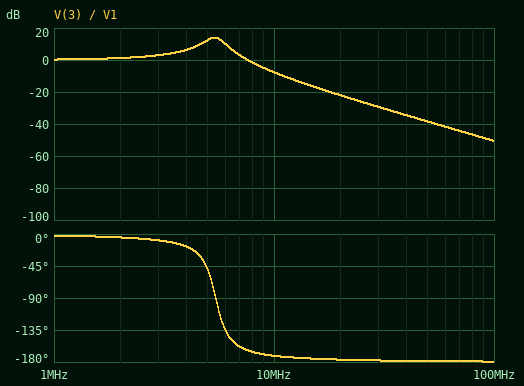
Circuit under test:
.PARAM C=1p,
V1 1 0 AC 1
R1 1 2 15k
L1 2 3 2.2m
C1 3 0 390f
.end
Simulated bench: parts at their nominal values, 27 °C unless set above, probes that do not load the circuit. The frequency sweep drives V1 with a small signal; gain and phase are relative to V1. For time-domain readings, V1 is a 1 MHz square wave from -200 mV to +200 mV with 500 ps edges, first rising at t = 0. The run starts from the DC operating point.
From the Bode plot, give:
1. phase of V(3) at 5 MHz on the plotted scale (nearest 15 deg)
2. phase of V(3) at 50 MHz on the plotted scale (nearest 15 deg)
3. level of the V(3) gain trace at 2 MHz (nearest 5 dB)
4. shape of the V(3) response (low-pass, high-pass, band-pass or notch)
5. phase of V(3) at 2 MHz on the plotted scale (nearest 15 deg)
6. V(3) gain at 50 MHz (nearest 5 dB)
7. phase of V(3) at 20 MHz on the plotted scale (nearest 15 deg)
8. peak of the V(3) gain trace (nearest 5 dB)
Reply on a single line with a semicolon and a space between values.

-45 deg; -180 deg; 0 dB; low-pass; 0 deg; -40 dB; -180 deg; 15 dB
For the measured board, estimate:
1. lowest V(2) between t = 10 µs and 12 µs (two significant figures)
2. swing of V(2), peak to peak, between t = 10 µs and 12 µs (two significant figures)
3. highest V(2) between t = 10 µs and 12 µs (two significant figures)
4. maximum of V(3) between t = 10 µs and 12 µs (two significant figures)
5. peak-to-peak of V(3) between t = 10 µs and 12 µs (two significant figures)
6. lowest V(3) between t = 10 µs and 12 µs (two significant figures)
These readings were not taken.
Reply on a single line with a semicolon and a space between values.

-250 mV; 510 mV; 250 mV; 510 mV; 1.0 V; -510 mV
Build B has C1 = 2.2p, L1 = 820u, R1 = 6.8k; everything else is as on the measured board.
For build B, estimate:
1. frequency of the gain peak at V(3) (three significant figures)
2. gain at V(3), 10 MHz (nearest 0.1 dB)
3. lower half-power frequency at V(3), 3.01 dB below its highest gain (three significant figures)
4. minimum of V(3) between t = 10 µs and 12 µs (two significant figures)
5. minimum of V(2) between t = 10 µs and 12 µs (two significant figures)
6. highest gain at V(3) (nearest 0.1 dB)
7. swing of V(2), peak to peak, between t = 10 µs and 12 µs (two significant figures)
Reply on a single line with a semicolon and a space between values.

3.63 MHz; -15.8 dB; 2.88 MHz; -420 mV; -260 mV; 9.2 dB; 520 mV
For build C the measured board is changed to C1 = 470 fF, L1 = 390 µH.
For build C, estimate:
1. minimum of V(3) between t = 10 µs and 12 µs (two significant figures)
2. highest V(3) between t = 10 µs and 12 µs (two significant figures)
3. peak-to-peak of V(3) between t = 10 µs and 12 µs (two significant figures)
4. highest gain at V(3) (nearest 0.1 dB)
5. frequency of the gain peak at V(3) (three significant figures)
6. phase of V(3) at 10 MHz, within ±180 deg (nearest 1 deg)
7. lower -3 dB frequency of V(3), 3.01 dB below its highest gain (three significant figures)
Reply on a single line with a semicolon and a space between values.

-370 mV; 370 mV; 740 mV; 6.0 dB; 10.9 MHz; -58 deg; 7.07 MHz
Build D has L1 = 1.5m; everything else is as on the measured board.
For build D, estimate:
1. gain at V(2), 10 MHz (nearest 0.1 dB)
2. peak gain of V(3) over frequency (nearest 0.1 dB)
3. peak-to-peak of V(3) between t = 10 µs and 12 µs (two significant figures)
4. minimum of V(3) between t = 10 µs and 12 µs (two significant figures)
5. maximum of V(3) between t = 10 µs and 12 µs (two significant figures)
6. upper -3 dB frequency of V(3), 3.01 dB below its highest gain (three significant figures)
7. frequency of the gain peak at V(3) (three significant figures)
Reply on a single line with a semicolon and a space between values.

-0.3 dB; 12.4 dB; 940 mV; -470 mV; 470 mV; 7.24 MHz; 6.48 MHz
